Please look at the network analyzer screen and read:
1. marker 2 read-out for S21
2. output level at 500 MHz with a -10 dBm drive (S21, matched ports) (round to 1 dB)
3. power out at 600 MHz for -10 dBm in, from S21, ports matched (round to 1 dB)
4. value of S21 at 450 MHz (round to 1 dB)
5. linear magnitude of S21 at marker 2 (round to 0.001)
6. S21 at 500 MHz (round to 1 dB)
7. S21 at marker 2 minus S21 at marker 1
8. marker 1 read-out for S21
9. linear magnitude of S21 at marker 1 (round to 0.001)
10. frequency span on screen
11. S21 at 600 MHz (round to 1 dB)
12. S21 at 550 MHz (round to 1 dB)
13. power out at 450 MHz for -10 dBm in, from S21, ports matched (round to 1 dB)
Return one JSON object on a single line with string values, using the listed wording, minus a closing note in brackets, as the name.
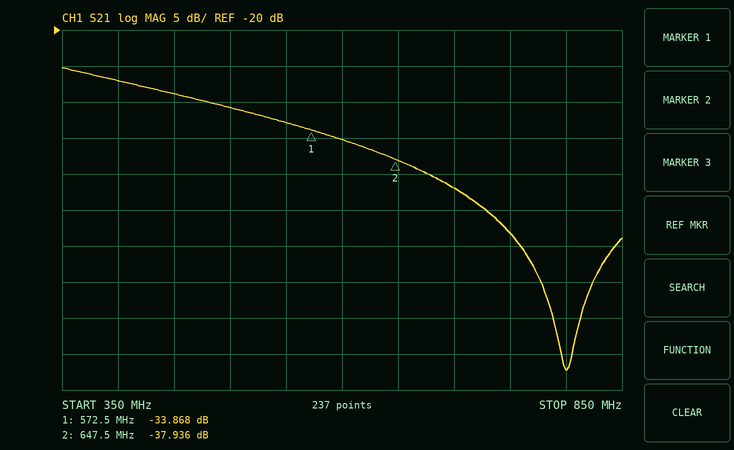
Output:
{"marker 2 read-out for S21": "-37.936 dB", "output level at 500 MHz with a -10 dBm drive (S21, matched ports)": "-41 dBm", "power out at 600 MHz for -10 dBm in, from S21, ports matched": "-45 dBm", "value of S21 at 450 MHz": "-29 dB", "linear magnitude of S21 at marker 2": "0.013", "S21 at 500 MHz": "-31 dB", "S21 at marker 2 minus S21 at marker 1": "-4.068 dB", "marker 1 read-out for S21": "-33.868 dB", "linear magnitude of S21 at marker 1": "0.020", "frequency span on screen": "500 MHz", "S21 at 600 MHz": "-35 dB", "S21 at 550 MHz": "-33 dB", "power out at 450 MHz for -10 dBm in, from S21, ports matched": "-39 dBm"}
